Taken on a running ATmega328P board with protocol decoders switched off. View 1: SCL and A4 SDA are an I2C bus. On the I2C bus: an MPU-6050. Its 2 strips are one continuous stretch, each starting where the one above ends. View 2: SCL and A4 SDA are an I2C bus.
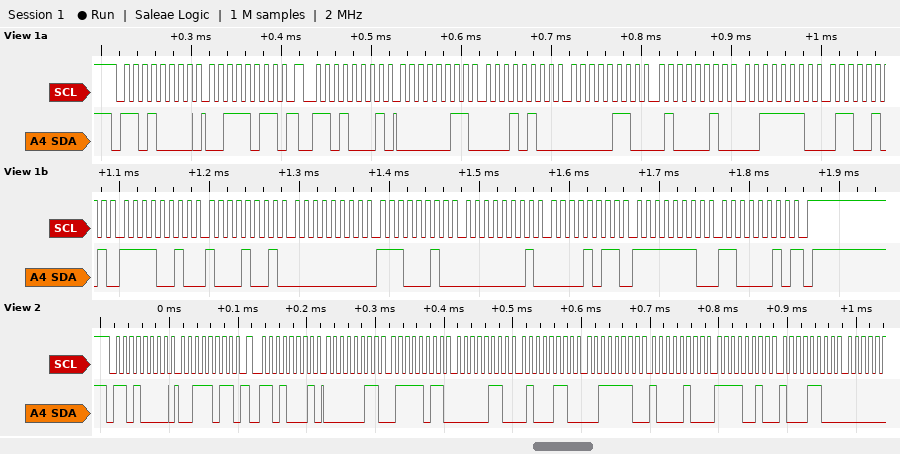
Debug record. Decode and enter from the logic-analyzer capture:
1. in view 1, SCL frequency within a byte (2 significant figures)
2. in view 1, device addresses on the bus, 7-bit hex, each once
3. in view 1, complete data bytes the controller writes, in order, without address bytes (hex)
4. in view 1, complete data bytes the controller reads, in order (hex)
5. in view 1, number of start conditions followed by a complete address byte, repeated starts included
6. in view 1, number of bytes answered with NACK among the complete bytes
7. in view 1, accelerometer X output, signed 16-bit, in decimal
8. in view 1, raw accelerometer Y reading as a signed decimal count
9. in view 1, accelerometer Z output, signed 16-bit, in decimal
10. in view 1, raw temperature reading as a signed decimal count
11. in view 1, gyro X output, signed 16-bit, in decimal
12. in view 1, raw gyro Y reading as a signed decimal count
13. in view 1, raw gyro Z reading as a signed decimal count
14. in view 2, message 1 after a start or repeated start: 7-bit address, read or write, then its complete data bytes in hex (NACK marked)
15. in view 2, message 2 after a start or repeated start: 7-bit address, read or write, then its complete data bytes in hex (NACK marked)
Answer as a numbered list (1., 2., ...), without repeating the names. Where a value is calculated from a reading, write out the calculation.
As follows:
1. 100 kHz
2. 0x68
3. 3B
4. 03 14 06 42 3E 65 F2 89 00 E2 01 0B FE C2
5. 2
6. 1
7. 0x0314 = 788
8. 0x0642 = 1602
9. 0x3E65 = 15973
10. 0xF289 = -3447
11. 0x00E2 = 226
12. 0x010B = 267
13. 0xFEC2 = -318
14. 0x68 write: 3B
15. 0x68 read: 03 7B 06 46 3E 84 F2 8C
